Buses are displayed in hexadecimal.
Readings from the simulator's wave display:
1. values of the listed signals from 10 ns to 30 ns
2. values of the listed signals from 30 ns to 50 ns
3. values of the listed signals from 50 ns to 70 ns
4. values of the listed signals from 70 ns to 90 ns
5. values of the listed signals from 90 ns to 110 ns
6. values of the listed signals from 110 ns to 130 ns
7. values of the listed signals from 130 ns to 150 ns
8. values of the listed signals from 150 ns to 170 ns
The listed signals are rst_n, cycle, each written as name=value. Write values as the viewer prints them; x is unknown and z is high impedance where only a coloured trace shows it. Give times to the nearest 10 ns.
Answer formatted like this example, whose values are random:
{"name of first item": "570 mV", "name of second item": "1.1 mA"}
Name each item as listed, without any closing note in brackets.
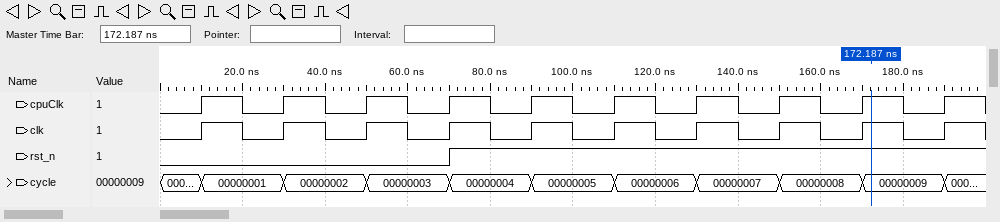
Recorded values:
{"values of the listed signals from 10 ns to 30 ns": "rst_n=0, cycle=00000001", "values of the listed signals from 30 ns to 50 ns": "rst_n=0, cycle=00000002", "values of the listed signals from 50 ns to 70 ns": "rst_n=0, cycle=00000003", "values of the listed signals from 70 ns to 90 ns": "rst_n=1, cycle=00000004", "values of the listed signals from 90 ns to 110 ns": "rst_n=1, cycle=00000005", "values of the listed signals from 110 ns to 130 ns": "rst_n=1, cycle=00000006", "values of the listed signals from 130 ns to 150 ns": "rst_n=1, cycle=00000007", "values of the listed signals from 150 ns to 170 ns": "rst_n=1, cycle=00000008"}
